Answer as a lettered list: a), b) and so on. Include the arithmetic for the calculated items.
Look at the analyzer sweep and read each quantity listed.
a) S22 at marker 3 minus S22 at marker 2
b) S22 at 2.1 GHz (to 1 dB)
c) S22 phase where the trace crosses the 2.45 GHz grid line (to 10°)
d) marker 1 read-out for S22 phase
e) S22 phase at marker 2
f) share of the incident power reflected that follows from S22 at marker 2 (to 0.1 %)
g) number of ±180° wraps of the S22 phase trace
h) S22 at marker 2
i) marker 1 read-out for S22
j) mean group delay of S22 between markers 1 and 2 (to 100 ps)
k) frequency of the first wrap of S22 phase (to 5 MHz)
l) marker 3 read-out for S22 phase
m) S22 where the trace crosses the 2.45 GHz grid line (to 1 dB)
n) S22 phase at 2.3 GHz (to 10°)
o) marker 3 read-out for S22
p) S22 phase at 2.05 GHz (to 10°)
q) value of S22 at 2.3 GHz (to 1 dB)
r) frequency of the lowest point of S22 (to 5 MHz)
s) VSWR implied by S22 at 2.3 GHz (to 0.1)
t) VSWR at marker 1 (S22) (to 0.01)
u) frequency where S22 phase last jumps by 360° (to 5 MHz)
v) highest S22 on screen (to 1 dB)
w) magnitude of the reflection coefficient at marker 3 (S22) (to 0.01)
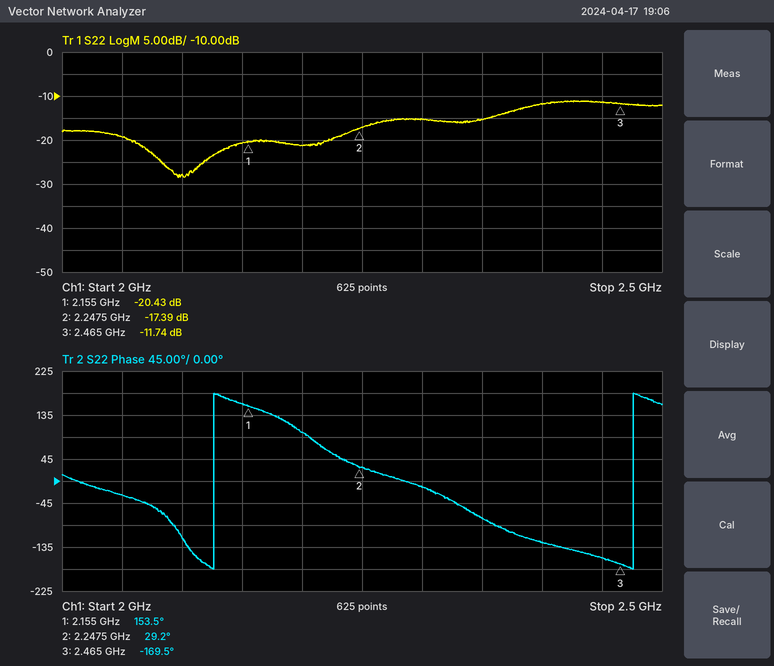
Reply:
a) -11.74 − (-17.39) = 5.65 dB
b) -28 dB
c) -160°
d) 153.5°
e) 29.2°
f) 10^(-17.39/10) ≈ 1.8 %
g) 2
h) -17.39 dB
i) -20.43 dB
j) −(29.2° − (153.5°))/(360° × 92.5 MHz) ≈ 3.7 ns
k) 2.125 GHz
l) -169.5°
m) -11 dB
n) -10°
o) -11.74 dB
p) -30°
q) -15 dB
r) 2.095 GHz
s) |Γ| = 10^(-15/20) = 0.1778; VSWR = (1 + 0.1778)/(1 − 0.1778) ≈ 1.4
t) (1 + 0.0952)/(1 − 0.0952) ≈ 1.21
u) 2.475 GHz
v) -11 dB
w) 10^(-11.74/20) ≈ 0.26
